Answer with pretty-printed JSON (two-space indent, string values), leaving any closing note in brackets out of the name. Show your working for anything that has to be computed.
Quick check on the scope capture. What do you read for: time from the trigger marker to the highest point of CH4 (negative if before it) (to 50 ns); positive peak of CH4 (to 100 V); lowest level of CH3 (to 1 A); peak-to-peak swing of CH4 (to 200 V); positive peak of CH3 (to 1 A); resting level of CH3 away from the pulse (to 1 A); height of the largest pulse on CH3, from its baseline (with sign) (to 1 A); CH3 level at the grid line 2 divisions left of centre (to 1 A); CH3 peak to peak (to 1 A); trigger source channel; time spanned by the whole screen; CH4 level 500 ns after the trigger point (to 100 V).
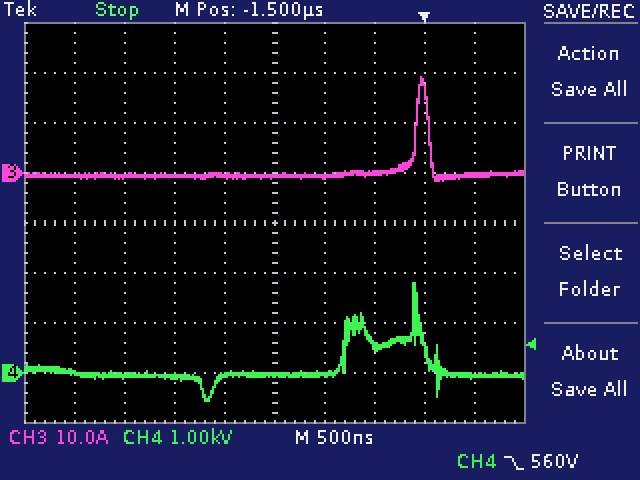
{
  "time from the trigger marker to the highest point of CH4 (negative if before it)": "-100 ns",
  "positive peak of CH4": "1.8 kV",
  "lowest level of CH3": "-2 A",
  "peak-to-peak swing of CH4": "2.4 kV",
  "positive peak of CH3": "19 A",
  "resting level of CH3 away from the pulse": "-1 A",
  "height of the largest pulse on CH3, from its baseline (with sign)": "19 A − (-1 A) = +20 A",
  "CH3 level at the grid line 2 divisions left of centre": "-1 A",
  "CH3 peak to peak": "19 A − (-2 A) = 21 A",
  "trigger source channel": "CH4",
  "time spanned by the whole screen": "5 µs",
  "CH4 level 500 ns after the trigger point": "-100 V"
}
